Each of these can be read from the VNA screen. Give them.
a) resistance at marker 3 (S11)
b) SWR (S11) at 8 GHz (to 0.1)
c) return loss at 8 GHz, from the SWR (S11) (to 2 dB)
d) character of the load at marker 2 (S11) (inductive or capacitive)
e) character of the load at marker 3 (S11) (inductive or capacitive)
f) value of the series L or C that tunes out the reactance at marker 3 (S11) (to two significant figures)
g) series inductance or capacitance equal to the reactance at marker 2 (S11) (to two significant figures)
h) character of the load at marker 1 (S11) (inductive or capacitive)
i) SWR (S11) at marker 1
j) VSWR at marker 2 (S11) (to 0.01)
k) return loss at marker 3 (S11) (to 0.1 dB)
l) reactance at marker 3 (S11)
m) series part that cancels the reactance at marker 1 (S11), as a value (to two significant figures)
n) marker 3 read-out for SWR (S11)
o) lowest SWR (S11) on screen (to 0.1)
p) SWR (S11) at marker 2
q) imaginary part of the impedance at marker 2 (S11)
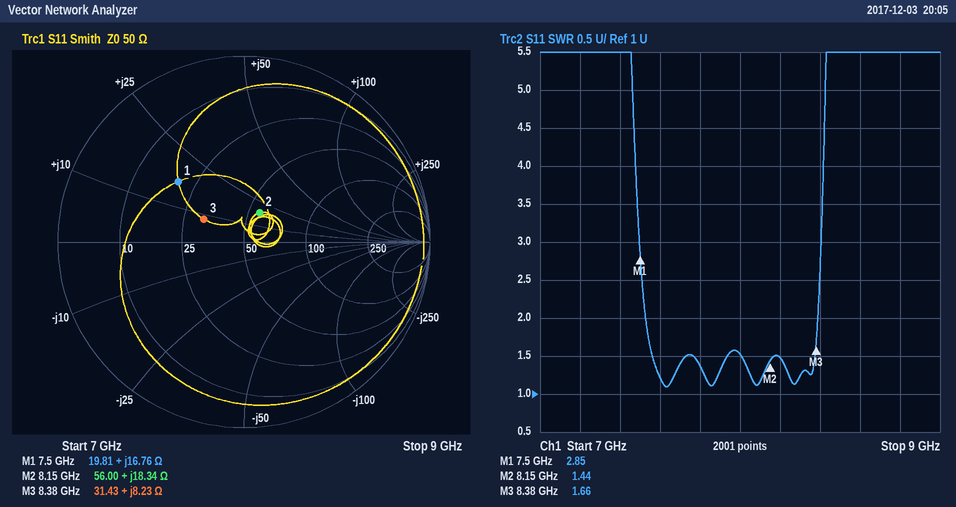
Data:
31.43 Ω
1.5
14 dB
inductive
inductive
2.3 pF
360 pH
inductive
2.85
1.44
12.1 dB
+8.23 Ω
1.3 pF
1.66
1.1
1.44
+18.34 Ω
